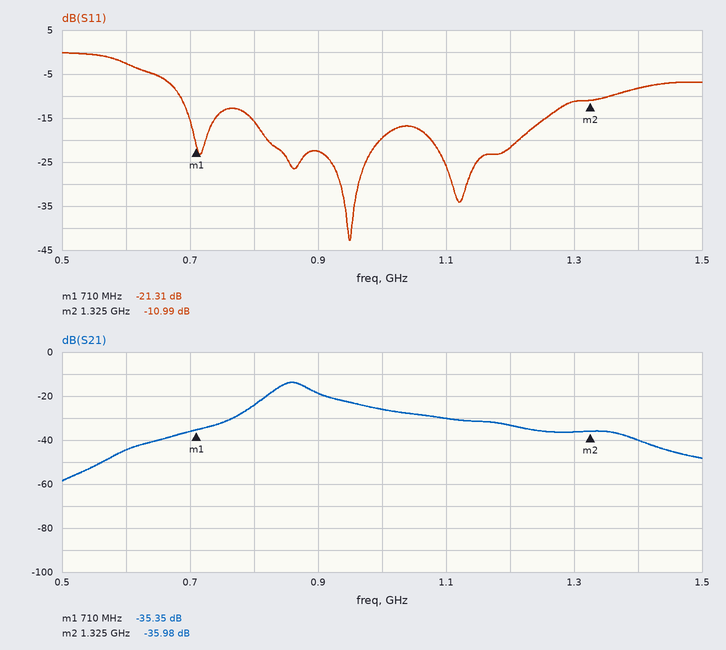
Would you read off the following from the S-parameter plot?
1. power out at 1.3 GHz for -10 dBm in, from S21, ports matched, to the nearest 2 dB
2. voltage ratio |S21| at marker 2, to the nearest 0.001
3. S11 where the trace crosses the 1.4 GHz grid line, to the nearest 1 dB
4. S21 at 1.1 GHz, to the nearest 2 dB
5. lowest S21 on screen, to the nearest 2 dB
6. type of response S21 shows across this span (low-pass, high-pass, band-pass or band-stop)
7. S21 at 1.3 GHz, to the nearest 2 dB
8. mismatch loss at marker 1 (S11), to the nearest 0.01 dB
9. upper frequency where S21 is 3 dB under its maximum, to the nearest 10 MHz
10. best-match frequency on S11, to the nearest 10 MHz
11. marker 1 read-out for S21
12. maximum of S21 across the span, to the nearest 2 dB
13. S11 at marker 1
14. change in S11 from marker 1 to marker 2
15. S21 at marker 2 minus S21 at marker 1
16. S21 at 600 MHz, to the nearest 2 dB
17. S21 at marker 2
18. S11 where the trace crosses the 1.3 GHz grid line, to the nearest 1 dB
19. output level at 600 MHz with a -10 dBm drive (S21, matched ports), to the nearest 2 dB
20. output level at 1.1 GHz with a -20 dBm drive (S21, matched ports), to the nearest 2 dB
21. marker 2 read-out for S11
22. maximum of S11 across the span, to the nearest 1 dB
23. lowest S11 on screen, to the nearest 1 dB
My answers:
-46 dBm
0.016
-8 dB
-30 dB
-58 dB
band-pass
-36 dB
0.03 dB
890 MHz
950 MHz
-35.35 dB
-14 dB
-21.31 dB
10.32 dB
-0.63 dB
-44 dB
-35.98 dB
-11 dB
-54 dBm
-50 dBm
-10.99 dB
0 dB
-43 dB
